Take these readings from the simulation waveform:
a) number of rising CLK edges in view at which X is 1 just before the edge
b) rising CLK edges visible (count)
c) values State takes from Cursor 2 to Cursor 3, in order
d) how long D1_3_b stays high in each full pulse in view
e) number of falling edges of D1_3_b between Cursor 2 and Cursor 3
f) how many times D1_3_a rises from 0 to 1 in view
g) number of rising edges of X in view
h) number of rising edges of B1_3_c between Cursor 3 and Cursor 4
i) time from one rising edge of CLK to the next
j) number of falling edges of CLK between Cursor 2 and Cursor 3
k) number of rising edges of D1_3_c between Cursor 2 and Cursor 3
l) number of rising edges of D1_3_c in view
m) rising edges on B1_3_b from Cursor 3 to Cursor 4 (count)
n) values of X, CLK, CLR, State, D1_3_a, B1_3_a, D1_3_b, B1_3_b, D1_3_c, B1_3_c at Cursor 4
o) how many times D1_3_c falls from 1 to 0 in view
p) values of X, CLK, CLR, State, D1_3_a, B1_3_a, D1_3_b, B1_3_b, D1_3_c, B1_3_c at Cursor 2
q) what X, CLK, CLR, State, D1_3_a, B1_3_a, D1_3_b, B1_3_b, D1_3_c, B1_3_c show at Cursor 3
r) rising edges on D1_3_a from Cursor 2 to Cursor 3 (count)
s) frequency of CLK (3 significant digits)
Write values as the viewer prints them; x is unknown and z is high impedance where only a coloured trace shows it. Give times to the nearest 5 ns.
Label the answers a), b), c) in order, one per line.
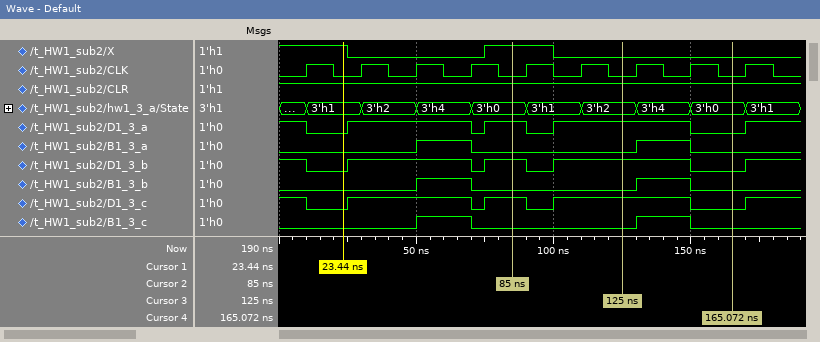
a) 2
b) 9
c) 3'h0, 3'h1, 3'h2
d) 45 ns, 15 ns, 50 ns
e) 1
f) 4
g) 1
h) 1
i) 20 ns
j) 2
k) 1
l) 4
m) 1
n) X=0, CLK=0, CLR=1, State=3'h0, D1_3_a=0, B1_3_a=0, D1_3_b=0, B1_3_b=0, D1_3_c=0, B1_3_c=0
o) 4
p) X=1, CLK=0, CLR=1, State=3'h0, D1_3_a=1, B1_3_a=0, D1_3_b=1, B1_3_b=0, D1_3_c=1, B1_3_c=0
q) X=0, CLK=0, CLR=1, State=3'h2, D1_3_a=1, B1_3_a=0, D1_3_b=1, B1_3_b=0, D1_3_c=1, B1_3_c=0
r) 1
s) 50.0 MHz
